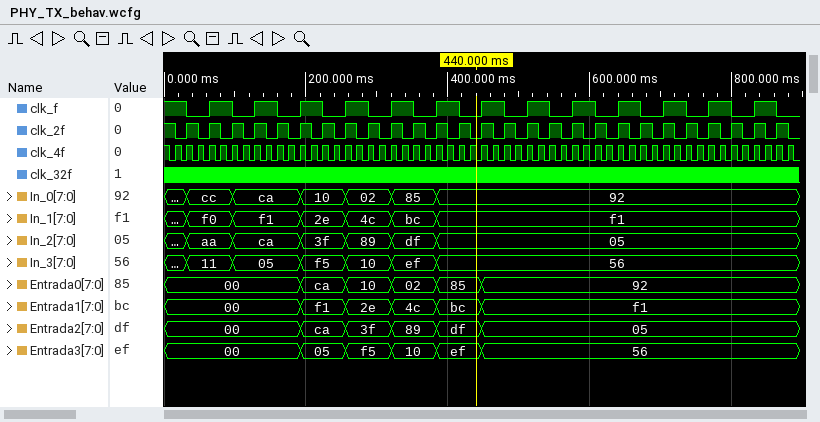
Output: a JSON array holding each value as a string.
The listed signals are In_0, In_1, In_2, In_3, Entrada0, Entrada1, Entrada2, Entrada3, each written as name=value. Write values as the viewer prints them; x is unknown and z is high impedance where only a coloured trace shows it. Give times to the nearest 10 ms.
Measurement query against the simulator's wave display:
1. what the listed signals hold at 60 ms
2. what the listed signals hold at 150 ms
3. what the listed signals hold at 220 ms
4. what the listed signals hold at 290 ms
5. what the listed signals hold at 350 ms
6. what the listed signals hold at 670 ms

["In_0=cc, In_1=f0, In_2=aa, In_3=11, Entrada0=00, Entrada1=00, Entrada2=00, Entrada3=00", "In_0=ca, In_1=f1, In_2=ca, In_3=05, Entrada0=00, Entrada1=00, Entrada2=00, Entrada3=00", "In_0=10, In_1=2e, In_2=3f, In_3=f5, Entrada0=ca, Entrada1=f1, Entrada2=ca, Entrada3=05", "In_0=02, In_1=4c, In_2=89, In_3=10, Entrada0=10, Entrada1=2e, Entrada2=3f, Entrada3=f5", "In_0=85, In_1=bc, In_2=df, In_3=ef, Entrada0=02, Entrada1=4c, Entrada2=89, Entrada3=10", "In_0=92, In_1=f1, In_2=05, In_3=56, Entrada0=92, Entrada1=f1, Entrada2=05, Entrada3=56"]
